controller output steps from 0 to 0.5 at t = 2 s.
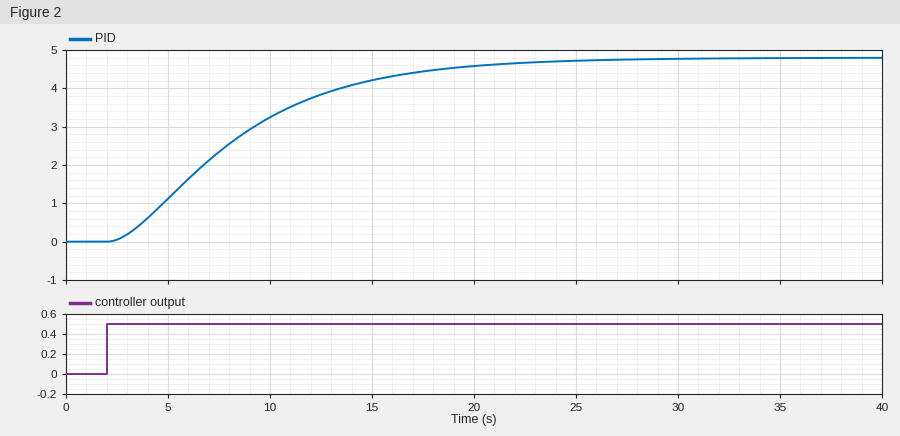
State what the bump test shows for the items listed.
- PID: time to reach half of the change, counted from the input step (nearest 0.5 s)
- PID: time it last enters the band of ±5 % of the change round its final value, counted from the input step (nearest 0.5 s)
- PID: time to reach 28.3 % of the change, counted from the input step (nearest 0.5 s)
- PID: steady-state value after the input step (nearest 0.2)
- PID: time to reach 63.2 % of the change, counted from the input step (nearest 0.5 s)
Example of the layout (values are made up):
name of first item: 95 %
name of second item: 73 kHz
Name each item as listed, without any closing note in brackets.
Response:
PID: time to reach half of the change, counted from the input step: 5.5 s
PID: time it last enters the band of ±5 % of the change round its final value, counted from the input step: 17.5 s
PID: time to reach 28.3 % of the change, counted from the input step: 3.5 s
PID: steady-state value after the input step: 4.8
PID: time to reach 63.2 % of the change, counted from the input step: 7.5 s
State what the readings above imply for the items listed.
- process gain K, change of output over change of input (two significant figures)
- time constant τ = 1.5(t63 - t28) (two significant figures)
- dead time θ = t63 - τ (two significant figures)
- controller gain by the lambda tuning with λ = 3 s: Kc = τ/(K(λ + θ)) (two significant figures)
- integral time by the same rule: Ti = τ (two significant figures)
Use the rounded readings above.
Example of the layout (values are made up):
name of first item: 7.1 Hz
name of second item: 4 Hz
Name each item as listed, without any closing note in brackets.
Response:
process gain K, change of output over change of input: 9.6
time constant τ = 1.5(t63 - t28): 6.0 s
dead time θ = t63 - τ: 1.5 s
controller gain by the lambda tuning with λ = 3 s: Kc = τ/(K(λ + θ)): 0.14
integral time by the same rule: Ti = τ: 6.0 s
